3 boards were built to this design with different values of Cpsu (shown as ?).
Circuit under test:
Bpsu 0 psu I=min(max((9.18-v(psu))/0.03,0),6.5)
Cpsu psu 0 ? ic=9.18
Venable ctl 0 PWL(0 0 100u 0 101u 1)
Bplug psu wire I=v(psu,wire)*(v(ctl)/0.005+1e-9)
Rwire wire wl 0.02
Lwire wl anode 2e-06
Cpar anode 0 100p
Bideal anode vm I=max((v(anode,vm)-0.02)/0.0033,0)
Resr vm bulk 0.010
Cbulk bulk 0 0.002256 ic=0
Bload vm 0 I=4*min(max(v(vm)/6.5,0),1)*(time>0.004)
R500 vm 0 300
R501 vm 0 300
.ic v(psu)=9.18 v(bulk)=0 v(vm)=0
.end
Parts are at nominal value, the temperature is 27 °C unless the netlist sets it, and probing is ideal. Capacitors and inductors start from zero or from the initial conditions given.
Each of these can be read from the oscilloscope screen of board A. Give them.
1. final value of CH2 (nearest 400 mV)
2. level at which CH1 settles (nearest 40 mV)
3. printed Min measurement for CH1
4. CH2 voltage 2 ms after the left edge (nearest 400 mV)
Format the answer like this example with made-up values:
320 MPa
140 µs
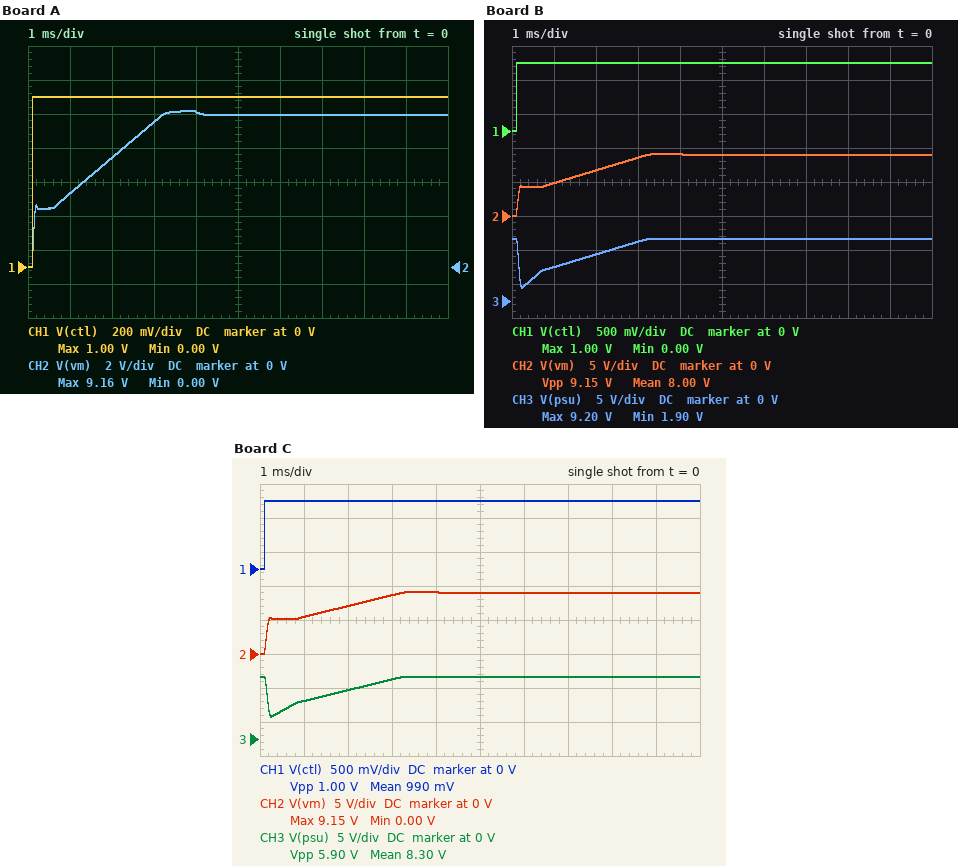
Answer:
8.8 V
1.00 V
0.00 V
6.4 V
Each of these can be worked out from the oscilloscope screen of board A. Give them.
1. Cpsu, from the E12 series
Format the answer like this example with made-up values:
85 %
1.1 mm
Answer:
820 µF
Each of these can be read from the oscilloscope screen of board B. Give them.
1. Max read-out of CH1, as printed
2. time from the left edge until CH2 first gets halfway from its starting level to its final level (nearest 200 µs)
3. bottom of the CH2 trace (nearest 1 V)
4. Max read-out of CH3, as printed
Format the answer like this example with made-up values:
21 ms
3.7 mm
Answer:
1.00 V
800 µs
0 V
9.20 V
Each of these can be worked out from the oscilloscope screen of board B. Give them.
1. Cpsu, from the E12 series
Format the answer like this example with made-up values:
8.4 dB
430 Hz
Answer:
1.2 mF
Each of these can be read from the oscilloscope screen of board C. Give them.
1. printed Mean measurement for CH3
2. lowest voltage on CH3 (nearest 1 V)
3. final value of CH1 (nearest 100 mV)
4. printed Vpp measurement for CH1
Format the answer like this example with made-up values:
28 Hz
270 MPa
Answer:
8.30 V
3 V
1.0 V
1.00 V
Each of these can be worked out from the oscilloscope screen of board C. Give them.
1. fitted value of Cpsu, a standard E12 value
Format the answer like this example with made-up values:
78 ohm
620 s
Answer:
1.8 mF
